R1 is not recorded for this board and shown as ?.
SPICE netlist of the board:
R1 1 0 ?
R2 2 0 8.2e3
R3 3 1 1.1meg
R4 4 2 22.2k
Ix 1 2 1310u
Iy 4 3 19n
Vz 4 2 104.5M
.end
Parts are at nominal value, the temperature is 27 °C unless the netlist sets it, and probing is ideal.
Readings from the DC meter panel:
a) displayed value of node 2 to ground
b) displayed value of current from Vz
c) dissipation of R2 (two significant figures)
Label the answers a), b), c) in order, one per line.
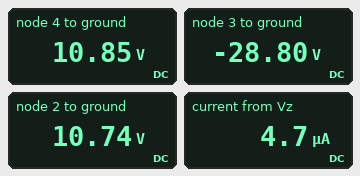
a) 10.74 V
b) 4.7 µA
c) 14 mW
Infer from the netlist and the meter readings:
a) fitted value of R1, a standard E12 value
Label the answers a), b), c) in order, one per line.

a) 22 kΩ
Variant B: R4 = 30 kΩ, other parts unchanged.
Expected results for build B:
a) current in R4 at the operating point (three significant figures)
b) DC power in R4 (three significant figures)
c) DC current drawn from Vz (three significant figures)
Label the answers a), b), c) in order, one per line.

a) 3.48 µA
b) 364 nW
c) 3.50 µA
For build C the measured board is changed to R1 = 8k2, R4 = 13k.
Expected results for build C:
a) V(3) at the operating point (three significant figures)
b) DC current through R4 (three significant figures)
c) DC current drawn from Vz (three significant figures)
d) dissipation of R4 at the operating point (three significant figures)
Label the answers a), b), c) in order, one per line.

a) -10.7 V
b) 8.04 µA
c) 8.06 µA
d) 840 nW
